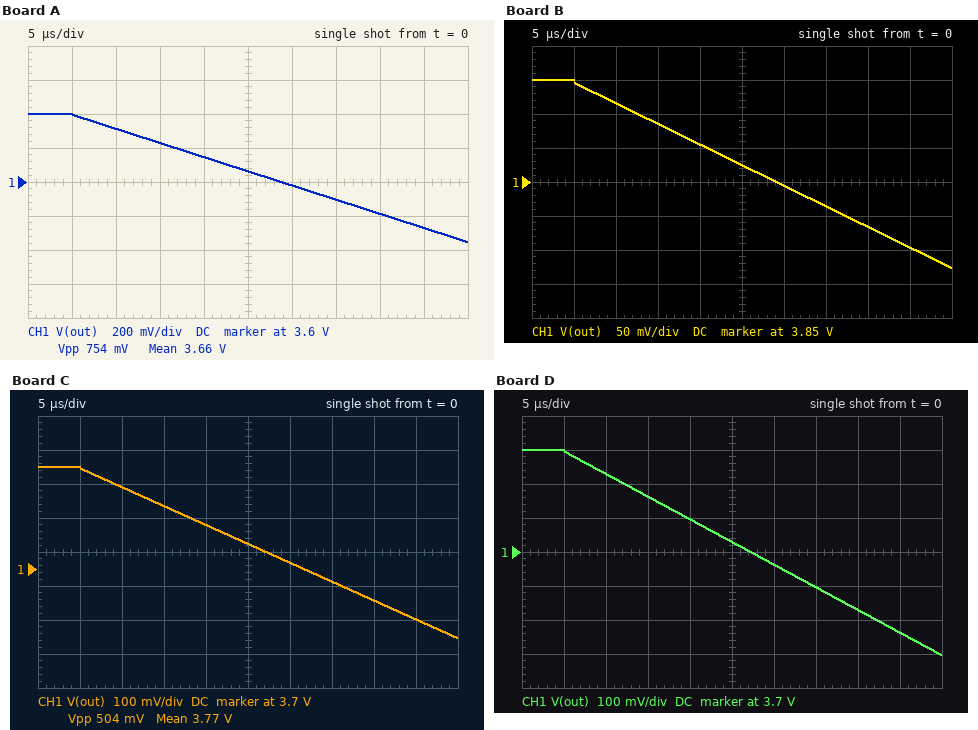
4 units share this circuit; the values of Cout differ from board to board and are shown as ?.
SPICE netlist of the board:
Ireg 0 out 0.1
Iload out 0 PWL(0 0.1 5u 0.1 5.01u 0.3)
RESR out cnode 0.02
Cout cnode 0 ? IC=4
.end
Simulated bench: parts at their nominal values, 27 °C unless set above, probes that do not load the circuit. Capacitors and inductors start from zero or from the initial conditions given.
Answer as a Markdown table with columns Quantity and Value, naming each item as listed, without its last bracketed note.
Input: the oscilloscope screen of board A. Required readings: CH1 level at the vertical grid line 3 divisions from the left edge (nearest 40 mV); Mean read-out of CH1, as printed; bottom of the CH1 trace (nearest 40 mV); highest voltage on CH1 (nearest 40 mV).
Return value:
| Quantity | Value |
|---|---|
| CH1 level at the vertical grid line 3 divisions from the left edge | 3.84 V |
| Mean read-out of CH1, as printed | 3.66 V |
| bottom of the CH1 trace | 3.24 V |
| highest voltage on CH1 | 4.00 V |
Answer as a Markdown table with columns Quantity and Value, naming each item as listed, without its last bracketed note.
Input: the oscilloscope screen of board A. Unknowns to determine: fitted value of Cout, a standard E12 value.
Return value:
| Quantity | Value |
|---|---|
| fitted value of Cout, a standard E12 value | 12 µF |
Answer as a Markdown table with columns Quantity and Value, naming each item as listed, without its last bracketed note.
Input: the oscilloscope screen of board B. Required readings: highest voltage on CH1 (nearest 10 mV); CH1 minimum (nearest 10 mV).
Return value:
| Quantity | Value |
|---|---|
| highest voltage on CH1 | 4.00 V |
| CH1 minimum | 3.72 V |
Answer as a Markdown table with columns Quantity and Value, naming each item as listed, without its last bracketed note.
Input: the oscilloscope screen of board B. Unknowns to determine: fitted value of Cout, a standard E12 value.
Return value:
| Quantity | Value |
|---|---|
| fitted value of Cout, a standard E12 value | 33 µF |
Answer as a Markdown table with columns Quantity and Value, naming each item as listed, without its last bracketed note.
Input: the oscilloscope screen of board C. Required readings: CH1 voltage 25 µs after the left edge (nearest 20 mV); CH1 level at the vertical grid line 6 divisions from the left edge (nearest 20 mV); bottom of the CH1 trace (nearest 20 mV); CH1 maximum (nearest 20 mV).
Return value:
| Quantity | Value |
|---|---|
| CH1 voltage 25 µs after the left edge | 3.78 V |
| CH1 level at the vertical grid line 6 divisions from the left edge | 3.72 V |
| bottom of the CH1 trace | 3.50 V |
| CH1 maximum | 4.00 V |
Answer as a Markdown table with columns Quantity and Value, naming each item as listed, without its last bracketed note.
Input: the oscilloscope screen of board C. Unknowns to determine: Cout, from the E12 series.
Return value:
| Quantity | Value |
|---|---|
| Cout, from the E12 series | 18 µF |
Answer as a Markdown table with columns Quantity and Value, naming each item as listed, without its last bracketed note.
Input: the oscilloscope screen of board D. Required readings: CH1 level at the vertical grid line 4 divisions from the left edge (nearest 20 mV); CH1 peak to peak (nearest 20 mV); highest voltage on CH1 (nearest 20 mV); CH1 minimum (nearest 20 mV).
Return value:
| Quantity | Value |
|---|---|
| CH1 level at the vertical grid line 4 divisions from the left edge | 3.80 V |
| CH1 peak to peak | 600 mV |
| highest voltage on CH1 | 4.00 V |
| CH1 minimum | 3.40 V |
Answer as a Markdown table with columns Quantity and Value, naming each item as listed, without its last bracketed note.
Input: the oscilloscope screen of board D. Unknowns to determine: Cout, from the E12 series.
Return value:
| Quantity | Value |
|---|---|
| Cout, from the E12 series | 15 µF |
